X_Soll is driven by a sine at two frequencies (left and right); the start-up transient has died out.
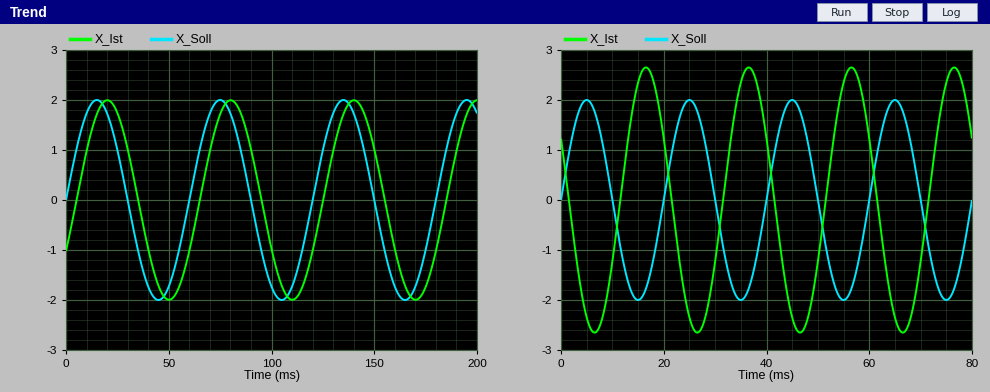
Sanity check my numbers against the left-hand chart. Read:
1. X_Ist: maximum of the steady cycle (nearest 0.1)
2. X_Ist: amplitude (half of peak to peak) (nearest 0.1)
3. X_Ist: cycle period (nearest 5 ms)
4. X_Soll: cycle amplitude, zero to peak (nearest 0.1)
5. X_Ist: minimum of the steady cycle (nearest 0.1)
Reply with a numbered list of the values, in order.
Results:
1. 2.0
2. 2.0
3. 60 ms
4. 2.0
5. -2.0
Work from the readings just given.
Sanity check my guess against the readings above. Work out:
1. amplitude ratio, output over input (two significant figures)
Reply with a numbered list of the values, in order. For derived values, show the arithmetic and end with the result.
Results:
1. 2 / 2 = 1.0
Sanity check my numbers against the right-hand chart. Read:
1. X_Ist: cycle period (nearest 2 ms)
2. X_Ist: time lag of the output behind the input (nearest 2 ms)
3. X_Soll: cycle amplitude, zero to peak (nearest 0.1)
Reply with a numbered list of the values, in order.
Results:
1. 20 ms
2. 12 ms
3. 2.0
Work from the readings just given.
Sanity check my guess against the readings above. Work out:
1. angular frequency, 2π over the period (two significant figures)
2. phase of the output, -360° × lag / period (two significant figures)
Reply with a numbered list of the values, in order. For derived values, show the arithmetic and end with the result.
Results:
1. 2π / 20 = 0.31 rad/ms
2. -360 × 12 / 20 = -220°
